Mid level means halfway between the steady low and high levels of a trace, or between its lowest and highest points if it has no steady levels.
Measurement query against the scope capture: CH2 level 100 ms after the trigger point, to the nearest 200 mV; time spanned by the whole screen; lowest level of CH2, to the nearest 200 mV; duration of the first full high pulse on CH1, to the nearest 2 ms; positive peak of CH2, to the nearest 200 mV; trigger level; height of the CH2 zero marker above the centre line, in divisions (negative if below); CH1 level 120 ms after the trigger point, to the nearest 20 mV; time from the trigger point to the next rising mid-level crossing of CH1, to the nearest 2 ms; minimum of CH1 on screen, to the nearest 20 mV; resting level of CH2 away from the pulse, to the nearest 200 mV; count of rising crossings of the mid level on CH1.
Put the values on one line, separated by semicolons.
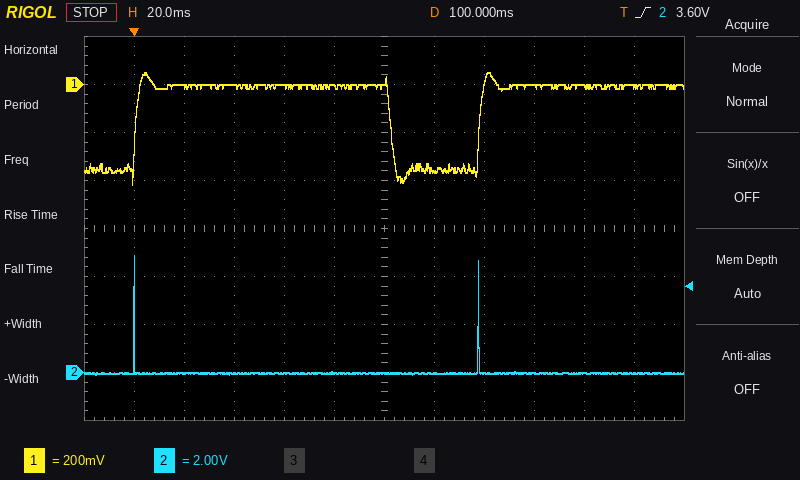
0.0 V; 240 ms; 0.0 V; 102 ms; 4.8 V; 3.60 V; -3.0 div; -360 mV; 138 ms; -420 mV; 0.0 V; 2
